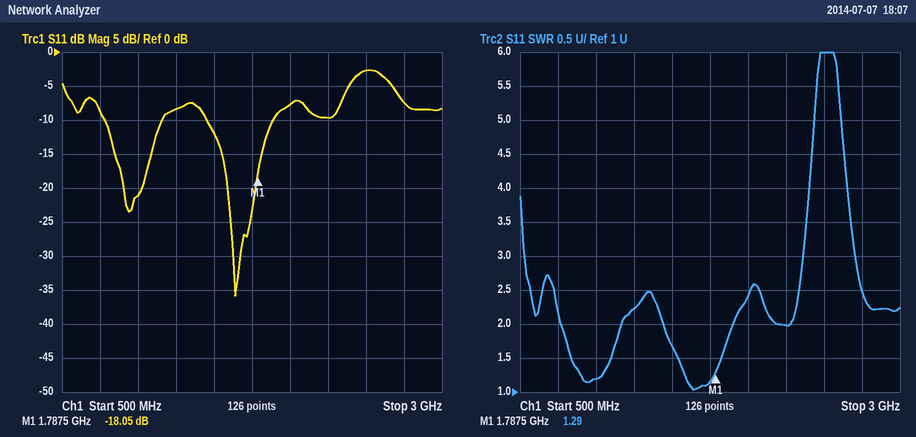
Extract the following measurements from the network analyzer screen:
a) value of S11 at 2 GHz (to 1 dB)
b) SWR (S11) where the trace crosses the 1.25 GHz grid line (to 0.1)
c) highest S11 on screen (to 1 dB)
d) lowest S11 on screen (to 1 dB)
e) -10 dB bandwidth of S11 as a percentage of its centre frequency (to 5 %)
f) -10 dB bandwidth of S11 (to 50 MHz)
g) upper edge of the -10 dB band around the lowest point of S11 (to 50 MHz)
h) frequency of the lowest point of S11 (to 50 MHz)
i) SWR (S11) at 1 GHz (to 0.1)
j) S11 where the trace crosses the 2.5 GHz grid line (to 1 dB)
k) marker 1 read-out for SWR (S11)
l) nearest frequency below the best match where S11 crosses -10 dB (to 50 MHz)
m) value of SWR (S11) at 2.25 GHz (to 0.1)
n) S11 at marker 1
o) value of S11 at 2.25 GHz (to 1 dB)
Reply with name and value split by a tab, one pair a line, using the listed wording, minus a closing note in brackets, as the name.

value of S11 at 2 GHz	-8 dB
SWR (S11) where the trace crosses the 1.25 GHz grid line	2.2
highest S11 on screen	-3 dB
lowest S11 on screen	-36 dB
-10 dB bandwidth of S11 as a percentage of its centre frequency	25 %
-10 dB bandwidth of S11	450 MHz
upper edge of the -10 dB band around the lowest point of S11	1.90 GHz
frequency of the lowest point of S11	1.65 GHz
SWR (S11) at 1 GHz	1.2
S11 where the trace crosses the 2.5 GHz grid line	-3 dB
marker 1 read-out for SWR	1.29
nearest frequency below the best match where S11 crosses -10 dB	1.45 GHz
value of SWR (S11) at 2.25 GHz	2.0
S11 at marker 1	-18.05 dB
value of S11 at 2.25 GHz	-10 dB
